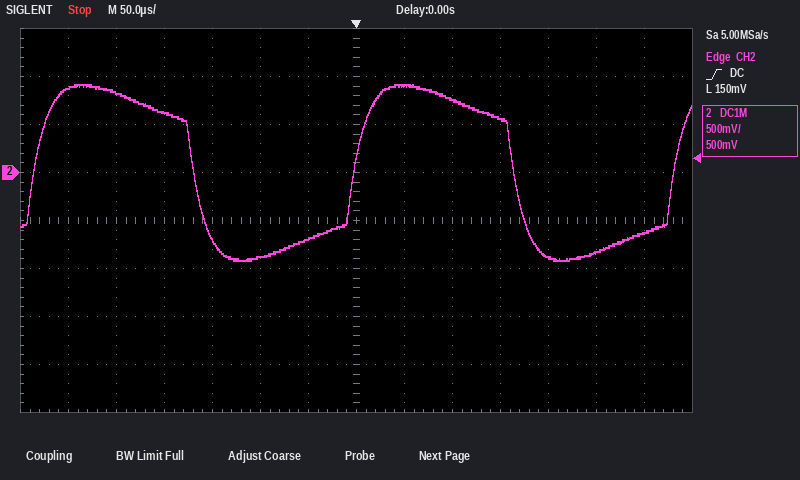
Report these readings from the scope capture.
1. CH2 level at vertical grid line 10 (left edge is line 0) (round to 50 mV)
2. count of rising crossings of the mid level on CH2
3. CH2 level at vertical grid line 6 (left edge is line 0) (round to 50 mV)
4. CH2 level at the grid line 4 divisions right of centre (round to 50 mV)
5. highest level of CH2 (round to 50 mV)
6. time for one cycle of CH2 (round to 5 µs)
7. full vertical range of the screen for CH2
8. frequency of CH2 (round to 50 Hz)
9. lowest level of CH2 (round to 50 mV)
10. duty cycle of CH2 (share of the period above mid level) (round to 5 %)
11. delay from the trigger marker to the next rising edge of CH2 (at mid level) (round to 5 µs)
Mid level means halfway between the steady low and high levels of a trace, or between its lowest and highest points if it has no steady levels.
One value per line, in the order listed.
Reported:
550 mV
3
-700 mV
-900 mV
900 mV
335 µs
4 V
3.00 kHz
-900 mV
50 %
330 µs
